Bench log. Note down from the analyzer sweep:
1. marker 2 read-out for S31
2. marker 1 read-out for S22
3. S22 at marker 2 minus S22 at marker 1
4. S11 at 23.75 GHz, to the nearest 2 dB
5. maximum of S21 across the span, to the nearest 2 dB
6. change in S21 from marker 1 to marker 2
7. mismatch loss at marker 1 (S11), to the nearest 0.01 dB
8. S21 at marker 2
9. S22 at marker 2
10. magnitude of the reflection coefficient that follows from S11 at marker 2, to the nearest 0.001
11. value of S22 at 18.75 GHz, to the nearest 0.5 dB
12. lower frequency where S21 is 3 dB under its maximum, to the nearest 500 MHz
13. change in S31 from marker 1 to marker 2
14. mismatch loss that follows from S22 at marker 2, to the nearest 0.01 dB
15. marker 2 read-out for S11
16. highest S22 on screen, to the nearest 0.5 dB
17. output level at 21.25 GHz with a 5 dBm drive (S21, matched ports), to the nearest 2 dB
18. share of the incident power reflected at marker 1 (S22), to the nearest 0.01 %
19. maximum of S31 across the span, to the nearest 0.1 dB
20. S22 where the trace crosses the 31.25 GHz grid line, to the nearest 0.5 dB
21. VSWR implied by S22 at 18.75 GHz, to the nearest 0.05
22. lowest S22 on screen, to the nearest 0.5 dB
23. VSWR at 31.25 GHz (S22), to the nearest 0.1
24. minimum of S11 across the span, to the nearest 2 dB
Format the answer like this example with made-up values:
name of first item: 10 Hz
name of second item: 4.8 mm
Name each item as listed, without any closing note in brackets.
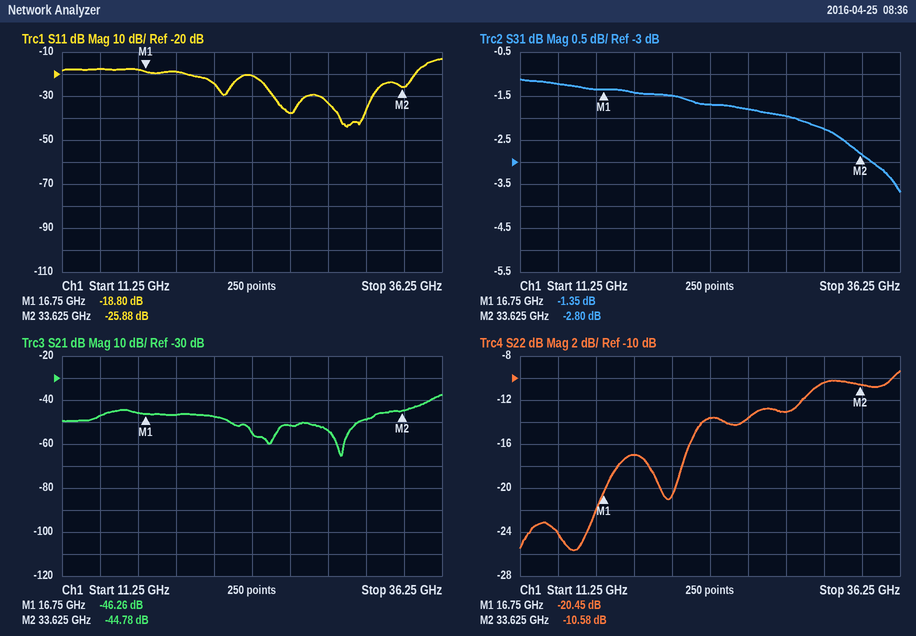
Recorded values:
marker 2 read-out for S31: -2.80 dB
marker 1 read-out for S22: -20.45 dB
S22 at marker 2 minus S22 at marker 1: 9.87 dB
S11 at 23.75 GHz, to the nearest 2 dB: -20 dB
maximum of S21 across the span, to the nearest 2 dB: -38 dB
change in S21 from marker 1 to marker 2: 1.48 dB
mismatch loss at marker 1 (S11), to the nearest 0.01 dB: 0.06 dB
S21 at marker 2: -44.78 dB
S22 at marker 2: -10.58 dB
magnitude of the reflection coefficient that follows from S11 at marker 2, to the nearest 0.001: 0.051
value of S22 at 18.75 GHz, to the nearest 0.5 dB: -17.0 dB
lower frequency where S21 is 3 dB under its maximum, to the nearest 500 MHz: 35.5 GHz
change in S31 from marker 1 to marker 2: -1.45 dB
mismatch loss that follows from S22 at marker 2, to the nearest 0.01 dB: 0.40 dB
marker 2 read-out for S11: -25.88 dB
highest S22 on screen, to the nearest 0.5 dB: -9.5 dB
output level at 21.25 GHz with a 5 dBm drive (S21, matched ports), to the nearest 2 dB: -42 dBm
share of the incident power reflected at marker 1 (S22), to the nearest 0.01 %: 0.90 %
maximum of S31 across the span, to the nearest 0.1 dB: -1.1 dB
S22 where the trace crosses the 31.25 GHz grid line, to the nearest 0.5 dB: -10.5 dB
VSWR implied by S22 at 18.75 GHz, to the nearest 0.05: 1.35
lowest S22 on screen, to the nearest 0.5 dB: -25.5 dB
VSWR at 31.25 GHz (S22), to the nearest 0.1: 1.9
minimum of S11 across the span, to the nearest 2 dB: -44 dB
